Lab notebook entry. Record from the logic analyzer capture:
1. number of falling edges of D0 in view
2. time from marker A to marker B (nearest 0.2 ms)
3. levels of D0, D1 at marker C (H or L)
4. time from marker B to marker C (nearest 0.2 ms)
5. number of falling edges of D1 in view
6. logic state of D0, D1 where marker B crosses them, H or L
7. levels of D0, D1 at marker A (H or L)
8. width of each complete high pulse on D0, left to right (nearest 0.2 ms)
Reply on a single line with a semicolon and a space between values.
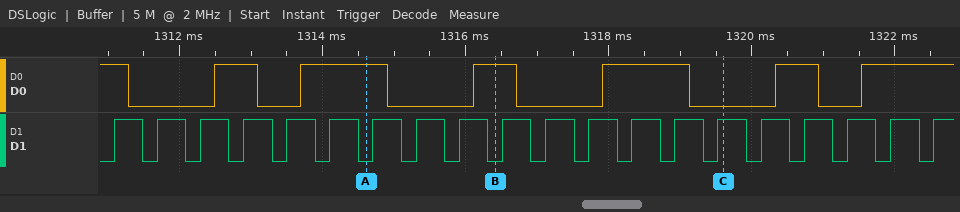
6; 1.8 ms; D0=L, D1=H; 3.2 ms; 19; D0=H, D1=L; D0=H, D1=L; 0.6 ms, 1.2 ms, 0.6 ms, 1.2 ms, 0.6 ms
